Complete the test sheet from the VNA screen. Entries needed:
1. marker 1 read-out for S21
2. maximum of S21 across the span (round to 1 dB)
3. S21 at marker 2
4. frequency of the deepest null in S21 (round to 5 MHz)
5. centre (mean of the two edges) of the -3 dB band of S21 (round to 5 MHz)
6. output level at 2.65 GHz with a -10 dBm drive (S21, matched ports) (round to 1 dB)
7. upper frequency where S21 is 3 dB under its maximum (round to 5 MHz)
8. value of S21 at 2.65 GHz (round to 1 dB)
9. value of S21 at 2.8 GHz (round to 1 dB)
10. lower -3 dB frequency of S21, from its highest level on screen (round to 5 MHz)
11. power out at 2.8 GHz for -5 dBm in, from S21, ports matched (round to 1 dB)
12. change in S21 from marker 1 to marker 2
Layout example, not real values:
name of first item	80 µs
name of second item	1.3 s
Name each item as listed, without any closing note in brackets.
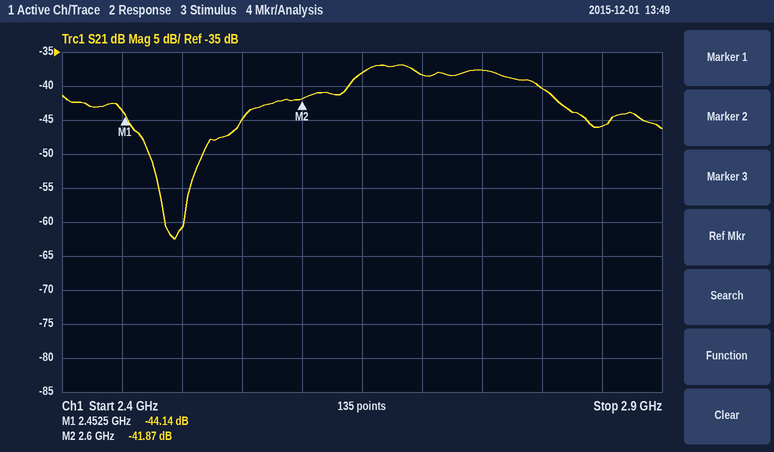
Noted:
marker 1 read-out for S21	-44.14 dB
maximum of S21 across the span	-37 dB
S21 at marker 2	-41.87 dB
frequency of the deepest null in S21	2.495 GHz
centre (mean of the two edges) of the -3 dB band of S21	2.720 GHz
output level at 2.65 GHz with a -10 dBm drive (S21, matched ports)	-48 dBm
upper frequency where S21 is 3 dB under its maximum	2.795 GHz
value of S21 at 2.65 GHz	-38 dB
value of S21 at 2.8 GHz	-40 dB
lower -3 dB frequency of S21, from its highest level on screen	2.640 GHz
power out at 2.8 GHz for -5 dBm in, from S21, ports matched	-45 dBm
change in S21 from marker 1 to marker 2	2.27 dB
